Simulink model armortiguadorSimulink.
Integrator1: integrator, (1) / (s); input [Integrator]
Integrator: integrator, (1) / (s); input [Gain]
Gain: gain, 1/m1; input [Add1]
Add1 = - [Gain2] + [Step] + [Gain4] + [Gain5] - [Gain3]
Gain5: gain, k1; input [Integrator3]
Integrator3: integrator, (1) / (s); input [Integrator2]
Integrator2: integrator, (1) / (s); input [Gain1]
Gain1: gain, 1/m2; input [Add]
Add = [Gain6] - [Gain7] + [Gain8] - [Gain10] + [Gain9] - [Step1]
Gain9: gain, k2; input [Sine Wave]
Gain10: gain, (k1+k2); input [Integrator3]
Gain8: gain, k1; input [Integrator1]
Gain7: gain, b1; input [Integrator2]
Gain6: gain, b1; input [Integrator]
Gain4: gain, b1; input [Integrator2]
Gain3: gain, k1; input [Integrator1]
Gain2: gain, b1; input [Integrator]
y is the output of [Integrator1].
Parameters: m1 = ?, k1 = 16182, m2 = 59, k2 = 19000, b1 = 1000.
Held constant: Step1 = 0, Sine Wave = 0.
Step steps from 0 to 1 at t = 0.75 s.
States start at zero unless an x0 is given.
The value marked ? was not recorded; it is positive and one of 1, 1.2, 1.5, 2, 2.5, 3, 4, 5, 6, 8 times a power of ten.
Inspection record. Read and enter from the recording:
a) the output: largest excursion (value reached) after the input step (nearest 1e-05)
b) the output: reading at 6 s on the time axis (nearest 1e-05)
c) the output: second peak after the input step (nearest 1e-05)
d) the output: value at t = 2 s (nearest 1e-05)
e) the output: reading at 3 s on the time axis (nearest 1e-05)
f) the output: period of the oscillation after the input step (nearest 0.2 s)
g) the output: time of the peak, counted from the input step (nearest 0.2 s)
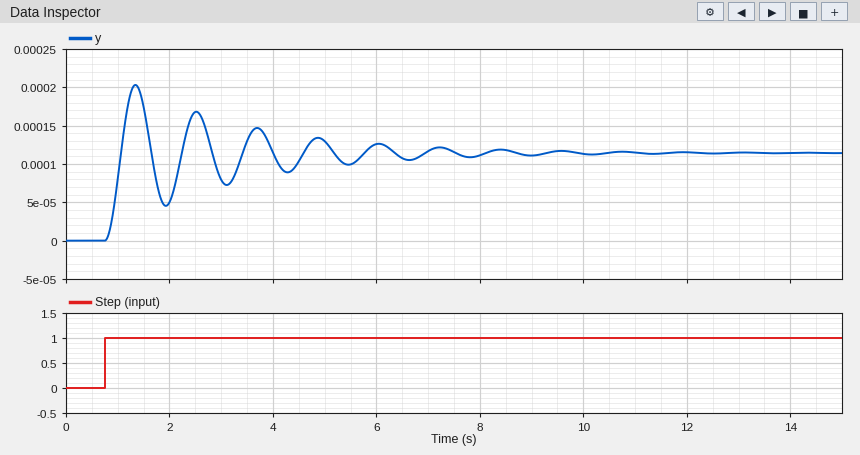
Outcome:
0.00020
0.00013
0.00017
0.00005
0.00008
1.2 s
0.6 s
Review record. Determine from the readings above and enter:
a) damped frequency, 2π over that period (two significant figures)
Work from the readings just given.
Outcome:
5.2 rad/s
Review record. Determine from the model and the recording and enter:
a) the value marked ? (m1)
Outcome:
300
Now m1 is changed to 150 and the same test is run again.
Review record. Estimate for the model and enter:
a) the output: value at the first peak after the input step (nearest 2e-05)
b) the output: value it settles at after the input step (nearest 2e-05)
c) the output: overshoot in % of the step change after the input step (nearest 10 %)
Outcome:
0.00020
0.00012
70 %
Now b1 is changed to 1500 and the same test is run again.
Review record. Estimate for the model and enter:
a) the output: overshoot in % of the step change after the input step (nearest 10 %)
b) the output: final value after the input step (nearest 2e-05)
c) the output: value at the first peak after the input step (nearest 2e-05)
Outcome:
70 %
0.00012
0.00020
